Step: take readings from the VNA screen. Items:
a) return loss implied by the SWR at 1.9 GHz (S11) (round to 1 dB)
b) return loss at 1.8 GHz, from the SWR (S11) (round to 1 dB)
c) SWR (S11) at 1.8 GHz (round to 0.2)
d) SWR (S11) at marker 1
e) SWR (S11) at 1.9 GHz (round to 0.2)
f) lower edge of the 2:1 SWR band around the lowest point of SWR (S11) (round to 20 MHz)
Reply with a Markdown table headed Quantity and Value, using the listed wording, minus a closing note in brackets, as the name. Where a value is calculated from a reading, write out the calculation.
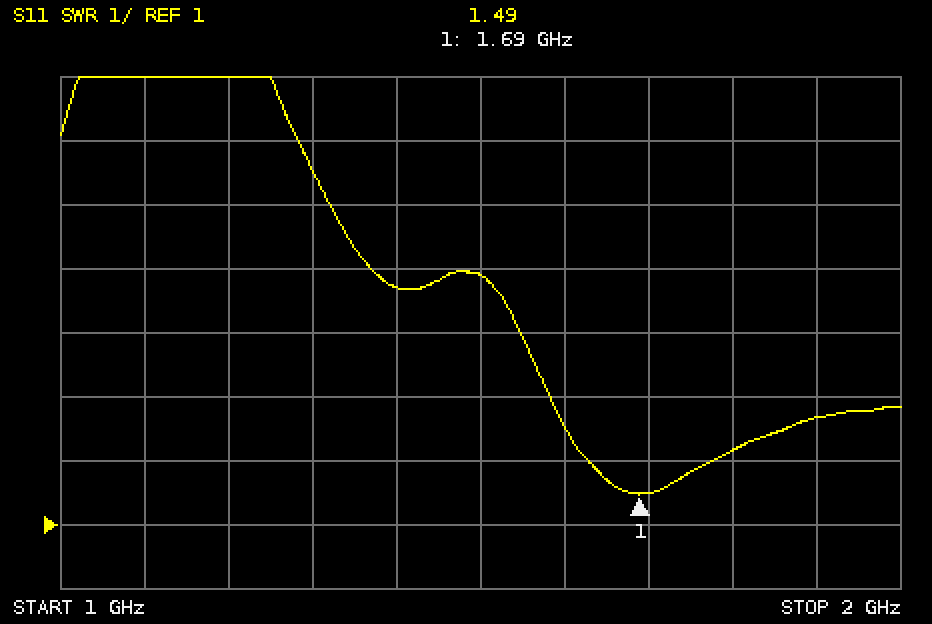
| Quantity | Value |
|---|---|
| return loss implied by the SWR at 1.9 GHz (S11) | −20 log10((2.6 − 1)/(2.6 + 1)) ≈ 7 dB |
| return loss at 1.8 GHz, from the SWR (S11) | −20 log10((2.2 − 1)/(2.2 + 1)) ≈ 9 dB |
| SWR (S11) at 1.8 GHz | 2.2 |
| SWR (S11) at marker 1 | 1.49 |
| SWR (S11) at 1.9 GHz | 2.6 |
| lower edge of the 2:1 SWR band around the lowest point of SWR (S11) | 1.62 GHz |
